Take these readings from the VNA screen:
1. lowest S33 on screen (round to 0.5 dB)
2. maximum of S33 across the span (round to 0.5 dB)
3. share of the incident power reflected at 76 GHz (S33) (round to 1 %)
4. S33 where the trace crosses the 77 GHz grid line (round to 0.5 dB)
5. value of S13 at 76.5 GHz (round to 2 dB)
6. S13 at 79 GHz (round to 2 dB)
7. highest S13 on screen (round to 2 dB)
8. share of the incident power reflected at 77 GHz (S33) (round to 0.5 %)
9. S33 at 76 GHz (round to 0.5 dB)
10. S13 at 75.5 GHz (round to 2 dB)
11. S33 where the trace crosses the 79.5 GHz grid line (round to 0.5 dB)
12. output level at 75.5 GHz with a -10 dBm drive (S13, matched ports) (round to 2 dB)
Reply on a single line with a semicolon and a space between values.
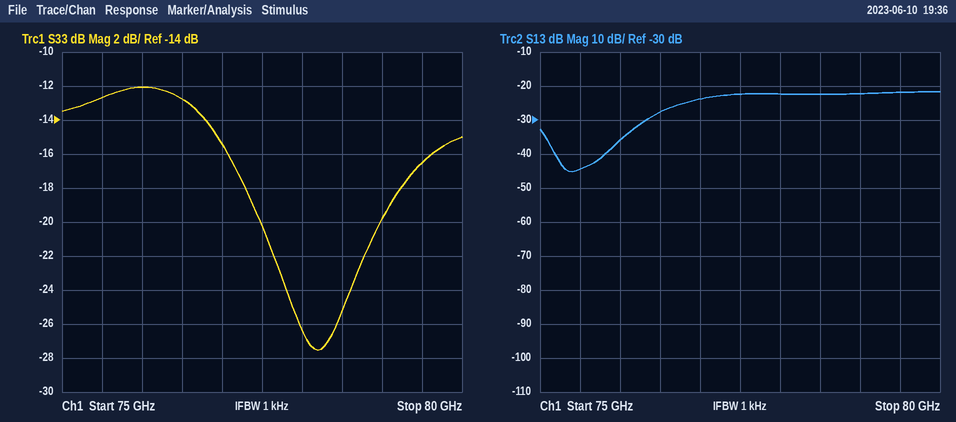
-27.5 dB; -12.0 dB; 6 %; -15.5 dB; -28 dB; -22 dB; -22 dB; 3.0 %; -12.0 dB; -44 dB; -16.5 dB; -54 dBm
